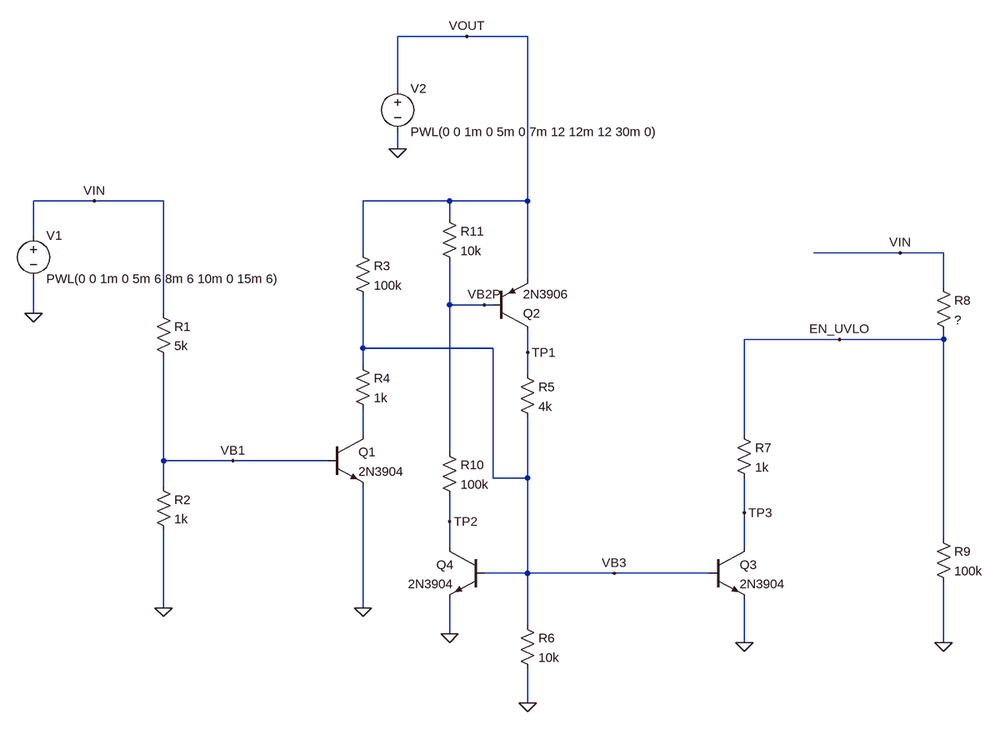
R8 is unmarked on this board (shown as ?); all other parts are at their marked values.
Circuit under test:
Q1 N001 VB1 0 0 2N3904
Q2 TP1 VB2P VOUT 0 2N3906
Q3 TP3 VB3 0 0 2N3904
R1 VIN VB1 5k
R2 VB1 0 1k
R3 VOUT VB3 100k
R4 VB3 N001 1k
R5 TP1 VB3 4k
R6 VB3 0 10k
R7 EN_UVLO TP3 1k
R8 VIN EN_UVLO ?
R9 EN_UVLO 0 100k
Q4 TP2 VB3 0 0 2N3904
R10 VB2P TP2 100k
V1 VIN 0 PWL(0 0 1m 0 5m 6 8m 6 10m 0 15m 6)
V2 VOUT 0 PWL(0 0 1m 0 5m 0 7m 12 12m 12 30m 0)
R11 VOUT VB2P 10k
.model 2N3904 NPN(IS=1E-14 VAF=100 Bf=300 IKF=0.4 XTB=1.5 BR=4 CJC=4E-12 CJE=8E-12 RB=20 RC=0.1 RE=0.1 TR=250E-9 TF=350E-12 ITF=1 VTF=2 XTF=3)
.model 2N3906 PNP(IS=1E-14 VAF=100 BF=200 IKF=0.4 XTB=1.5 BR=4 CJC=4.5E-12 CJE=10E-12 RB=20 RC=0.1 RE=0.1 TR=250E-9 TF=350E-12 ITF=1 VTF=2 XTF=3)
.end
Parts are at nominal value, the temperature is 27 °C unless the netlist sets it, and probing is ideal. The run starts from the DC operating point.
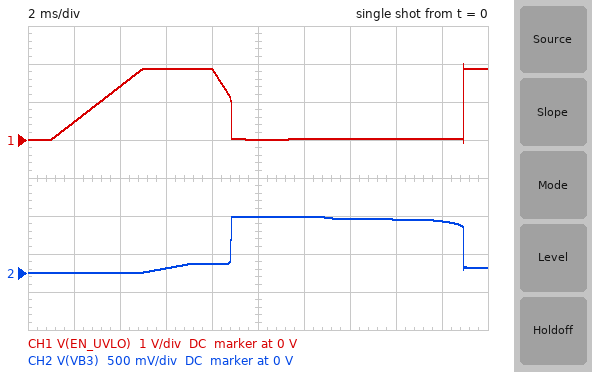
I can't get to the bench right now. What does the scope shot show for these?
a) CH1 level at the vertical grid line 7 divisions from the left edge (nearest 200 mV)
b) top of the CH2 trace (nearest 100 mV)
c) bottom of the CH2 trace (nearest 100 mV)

0 V
700 mV
0 V
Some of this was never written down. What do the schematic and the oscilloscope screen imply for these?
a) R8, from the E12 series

220 kΩ
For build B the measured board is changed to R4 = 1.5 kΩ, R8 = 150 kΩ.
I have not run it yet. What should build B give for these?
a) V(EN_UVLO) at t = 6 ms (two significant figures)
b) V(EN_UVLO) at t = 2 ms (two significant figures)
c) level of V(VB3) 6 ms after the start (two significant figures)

2.4 V
600 mV
83 mV
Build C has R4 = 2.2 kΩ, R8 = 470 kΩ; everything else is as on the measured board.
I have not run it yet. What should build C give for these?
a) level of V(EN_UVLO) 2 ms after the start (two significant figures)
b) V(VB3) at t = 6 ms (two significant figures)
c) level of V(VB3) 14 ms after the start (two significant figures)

260 mV
110 mV
720 mV
